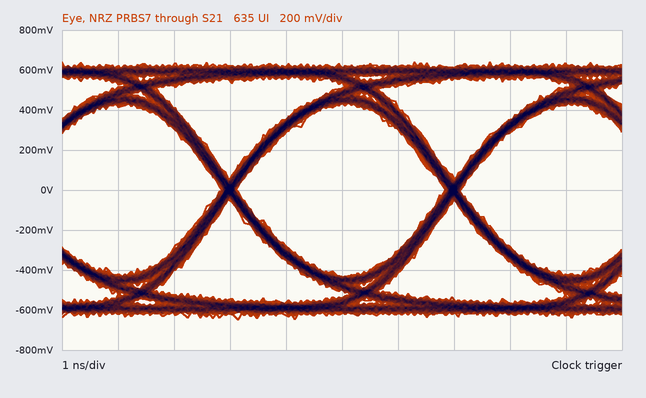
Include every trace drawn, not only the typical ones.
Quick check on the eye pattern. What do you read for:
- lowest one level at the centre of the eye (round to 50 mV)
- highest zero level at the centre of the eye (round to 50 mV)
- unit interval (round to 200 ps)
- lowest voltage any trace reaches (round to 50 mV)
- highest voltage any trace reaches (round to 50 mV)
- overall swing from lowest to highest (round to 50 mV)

450 mV
-450 mV
4.0 ns
-650 mV
650 mV
1.30 V
